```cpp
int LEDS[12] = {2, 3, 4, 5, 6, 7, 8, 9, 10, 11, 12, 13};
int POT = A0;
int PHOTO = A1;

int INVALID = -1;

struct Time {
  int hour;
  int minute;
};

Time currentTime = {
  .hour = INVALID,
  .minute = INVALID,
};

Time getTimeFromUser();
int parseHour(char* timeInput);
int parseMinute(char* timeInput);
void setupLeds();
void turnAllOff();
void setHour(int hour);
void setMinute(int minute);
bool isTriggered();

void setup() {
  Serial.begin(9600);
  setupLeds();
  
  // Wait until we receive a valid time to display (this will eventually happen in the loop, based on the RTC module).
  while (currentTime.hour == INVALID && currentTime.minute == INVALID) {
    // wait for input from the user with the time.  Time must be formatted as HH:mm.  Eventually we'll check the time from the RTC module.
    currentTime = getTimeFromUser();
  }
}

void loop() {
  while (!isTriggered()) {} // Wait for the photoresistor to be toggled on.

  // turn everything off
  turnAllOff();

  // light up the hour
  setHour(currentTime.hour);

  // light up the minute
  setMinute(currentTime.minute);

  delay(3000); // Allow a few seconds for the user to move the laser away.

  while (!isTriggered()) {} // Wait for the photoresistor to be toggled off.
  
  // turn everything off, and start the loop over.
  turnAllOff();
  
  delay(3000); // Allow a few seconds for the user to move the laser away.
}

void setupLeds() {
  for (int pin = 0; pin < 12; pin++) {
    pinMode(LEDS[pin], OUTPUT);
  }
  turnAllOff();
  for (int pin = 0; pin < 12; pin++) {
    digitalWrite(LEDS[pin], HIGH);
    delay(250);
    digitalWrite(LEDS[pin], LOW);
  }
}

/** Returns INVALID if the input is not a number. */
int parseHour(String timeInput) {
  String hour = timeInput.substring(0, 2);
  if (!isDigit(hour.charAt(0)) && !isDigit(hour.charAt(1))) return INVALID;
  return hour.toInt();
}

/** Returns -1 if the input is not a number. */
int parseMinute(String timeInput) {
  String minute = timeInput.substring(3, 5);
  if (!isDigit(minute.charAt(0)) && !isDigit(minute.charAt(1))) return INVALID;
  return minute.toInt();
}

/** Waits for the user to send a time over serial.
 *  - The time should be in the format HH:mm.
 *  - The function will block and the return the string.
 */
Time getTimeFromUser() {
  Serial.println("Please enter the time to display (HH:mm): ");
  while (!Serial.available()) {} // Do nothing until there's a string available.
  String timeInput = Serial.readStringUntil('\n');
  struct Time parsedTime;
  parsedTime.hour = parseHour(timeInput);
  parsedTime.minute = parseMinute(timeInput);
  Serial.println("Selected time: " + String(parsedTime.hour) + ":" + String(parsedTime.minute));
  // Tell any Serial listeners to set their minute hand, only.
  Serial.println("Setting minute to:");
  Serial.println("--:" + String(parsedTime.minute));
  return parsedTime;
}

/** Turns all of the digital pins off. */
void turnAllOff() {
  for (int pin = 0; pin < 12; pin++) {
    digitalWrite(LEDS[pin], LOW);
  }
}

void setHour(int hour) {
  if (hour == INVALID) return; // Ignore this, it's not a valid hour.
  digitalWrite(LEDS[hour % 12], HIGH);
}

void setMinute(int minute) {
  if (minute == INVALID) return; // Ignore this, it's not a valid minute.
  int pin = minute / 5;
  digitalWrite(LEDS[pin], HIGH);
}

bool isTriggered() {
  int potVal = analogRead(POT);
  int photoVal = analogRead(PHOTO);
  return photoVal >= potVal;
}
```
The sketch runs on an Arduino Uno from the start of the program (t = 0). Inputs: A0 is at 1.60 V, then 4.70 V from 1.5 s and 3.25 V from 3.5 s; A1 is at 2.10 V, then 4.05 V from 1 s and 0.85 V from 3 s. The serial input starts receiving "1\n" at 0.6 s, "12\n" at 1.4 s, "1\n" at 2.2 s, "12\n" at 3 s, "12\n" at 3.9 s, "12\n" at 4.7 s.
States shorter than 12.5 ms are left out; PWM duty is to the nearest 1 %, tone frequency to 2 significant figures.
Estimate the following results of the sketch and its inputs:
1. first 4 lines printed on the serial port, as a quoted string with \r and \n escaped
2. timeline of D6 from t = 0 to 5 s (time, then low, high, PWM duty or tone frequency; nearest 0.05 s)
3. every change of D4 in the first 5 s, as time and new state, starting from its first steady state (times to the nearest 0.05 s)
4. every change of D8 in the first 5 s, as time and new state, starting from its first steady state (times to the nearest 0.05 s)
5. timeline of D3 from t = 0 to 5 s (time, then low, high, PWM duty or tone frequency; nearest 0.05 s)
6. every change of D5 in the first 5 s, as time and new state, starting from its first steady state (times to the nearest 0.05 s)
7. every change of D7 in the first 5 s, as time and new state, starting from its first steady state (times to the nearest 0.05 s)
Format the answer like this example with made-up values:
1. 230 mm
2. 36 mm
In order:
1. "Please enter the time to display (HH:mm): \r\nSelected time: 1:-1\r\nSetting minute to:\r\n--:-1\r\n"
2. 0 s low; 1 s high; 1.25 s low
3. 0 s low; 0.5 s high; 0.75 s low
4. 0 s low; 1.5 s high; 1.75 s low
5. 0 s low; 0.25 s high; 0.5 s low
6. 0 s low; 0.75 s high; 1 s low
7. 0 s low; 1.25 s high; 1.5 s low
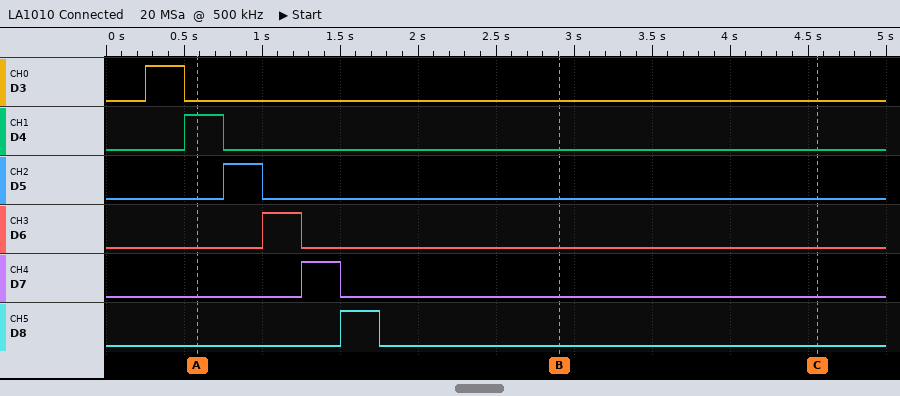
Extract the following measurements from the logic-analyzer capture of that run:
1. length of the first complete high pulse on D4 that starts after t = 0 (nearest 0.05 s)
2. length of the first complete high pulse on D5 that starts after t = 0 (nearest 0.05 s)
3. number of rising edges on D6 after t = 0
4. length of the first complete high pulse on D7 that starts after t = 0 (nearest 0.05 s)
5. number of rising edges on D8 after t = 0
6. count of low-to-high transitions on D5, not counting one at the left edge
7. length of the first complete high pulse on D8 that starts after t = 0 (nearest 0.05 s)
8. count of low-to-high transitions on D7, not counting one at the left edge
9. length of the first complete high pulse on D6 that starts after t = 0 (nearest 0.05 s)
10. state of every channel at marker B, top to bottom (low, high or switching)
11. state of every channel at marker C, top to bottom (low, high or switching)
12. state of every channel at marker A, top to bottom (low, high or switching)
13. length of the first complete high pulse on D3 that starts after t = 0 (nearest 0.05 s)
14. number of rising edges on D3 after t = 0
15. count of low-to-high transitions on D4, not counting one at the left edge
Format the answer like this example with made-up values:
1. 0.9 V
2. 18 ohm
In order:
1. 0.25 s
2. 0.25 s
3. 1
4. 0.25 s
5. 1
6. 1
7. 0.25 s
8. 1
9. 0.25 s
10. D3 low, D4 low, D5 low, D6 low, D7 low, D8 low
11. D3 low, D4 low, D5 low, D6 low, D7 low, D8 low
12. D3 low, D4 high, D5 low, D6 low, D7 low, D8 low
13. 0.25 s
14. 1
15. 1
